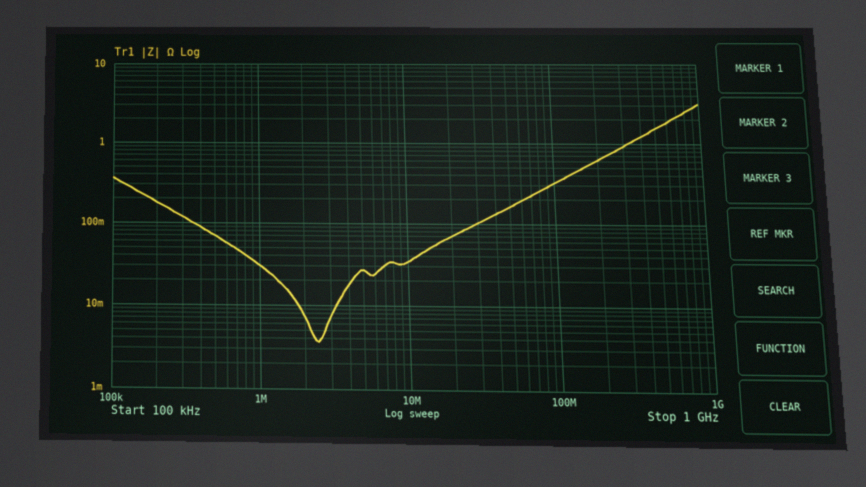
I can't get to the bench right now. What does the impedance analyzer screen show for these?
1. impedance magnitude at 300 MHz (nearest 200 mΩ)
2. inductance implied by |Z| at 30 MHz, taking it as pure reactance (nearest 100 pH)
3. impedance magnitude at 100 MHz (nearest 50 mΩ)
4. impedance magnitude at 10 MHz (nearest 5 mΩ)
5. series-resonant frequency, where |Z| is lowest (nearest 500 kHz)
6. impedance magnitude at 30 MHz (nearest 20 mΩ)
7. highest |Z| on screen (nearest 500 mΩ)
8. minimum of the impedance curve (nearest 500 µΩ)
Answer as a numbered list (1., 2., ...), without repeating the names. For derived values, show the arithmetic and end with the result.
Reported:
1. 1.0 Ω
2. L = 100 mΩ/(2π × 30 MHz) ≈ 531 pH, so 500 pH to the nearest 100 pH
3. 300 mΩ
4. 35 mΩ
5. 2.5 MHz
6. 100 mΩ
7. 3.0 Ω
8. 3.5 mΩ
